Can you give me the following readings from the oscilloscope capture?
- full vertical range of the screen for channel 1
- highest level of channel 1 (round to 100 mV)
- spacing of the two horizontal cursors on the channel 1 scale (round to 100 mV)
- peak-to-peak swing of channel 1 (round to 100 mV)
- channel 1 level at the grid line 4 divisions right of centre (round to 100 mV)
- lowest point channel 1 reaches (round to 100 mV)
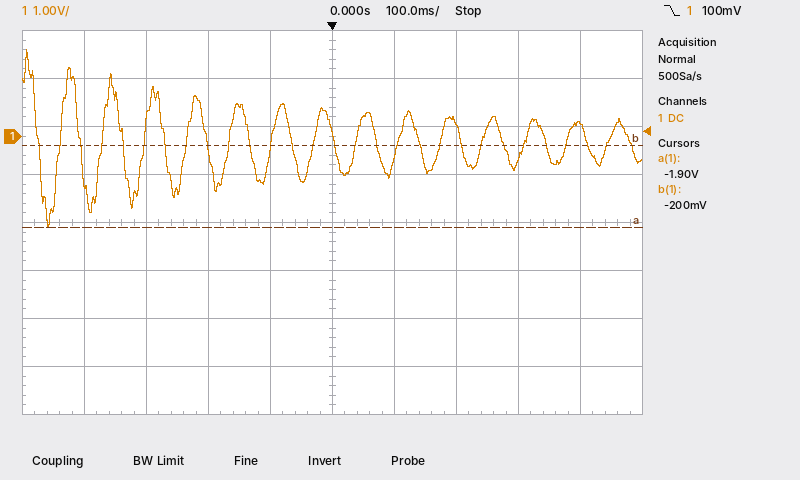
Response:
8 V
1.8 V
1.7 V
3.7 V
200 mV
-1.9 V
